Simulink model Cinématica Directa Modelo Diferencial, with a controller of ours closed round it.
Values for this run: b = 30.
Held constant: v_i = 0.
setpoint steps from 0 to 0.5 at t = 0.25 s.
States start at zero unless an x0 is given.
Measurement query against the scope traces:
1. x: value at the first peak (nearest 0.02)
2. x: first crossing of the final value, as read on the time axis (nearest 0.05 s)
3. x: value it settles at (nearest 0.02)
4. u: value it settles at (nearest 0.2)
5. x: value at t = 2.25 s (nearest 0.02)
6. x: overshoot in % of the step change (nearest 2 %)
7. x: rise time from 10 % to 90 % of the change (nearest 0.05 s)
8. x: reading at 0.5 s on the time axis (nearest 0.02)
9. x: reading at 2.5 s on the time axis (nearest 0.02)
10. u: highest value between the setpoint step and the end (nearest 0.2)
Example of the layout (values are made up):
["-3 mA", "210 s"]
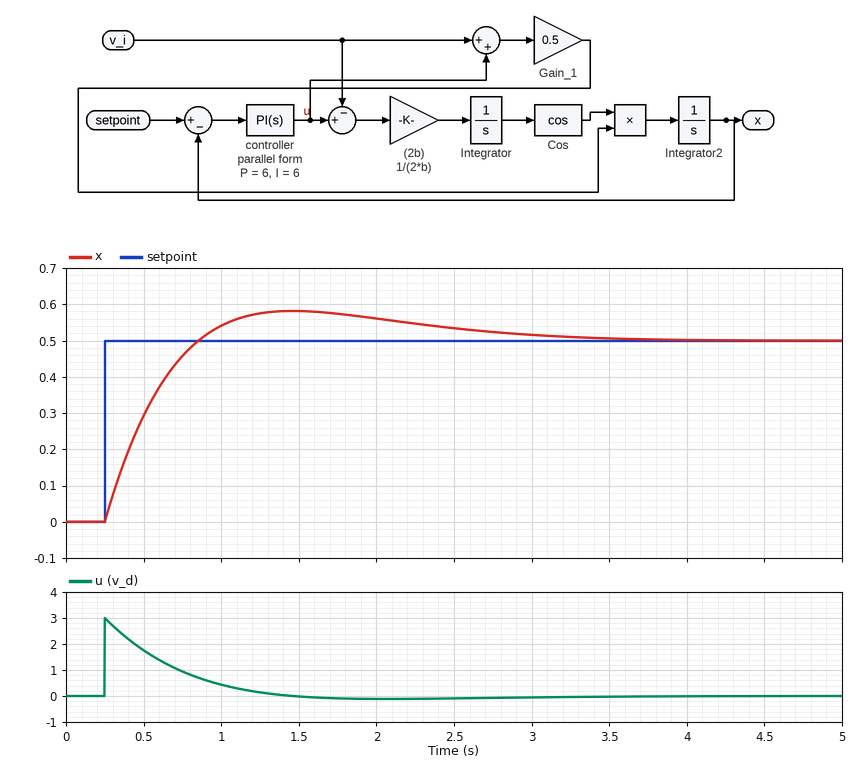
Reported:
["0.58", "0.85 s", "0.50", "0.0", "0.54", "16 %", "0.45 s", "0.30", "0.54", "3.0"]
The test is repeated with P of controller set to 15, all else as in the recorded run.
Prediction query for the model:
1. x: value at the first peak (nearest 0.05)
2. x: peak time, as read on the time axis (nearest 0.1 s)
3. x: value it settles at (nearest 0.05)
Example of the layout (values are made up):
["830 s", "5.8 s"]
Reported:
["0.50", "1.1 s", "0.50"]
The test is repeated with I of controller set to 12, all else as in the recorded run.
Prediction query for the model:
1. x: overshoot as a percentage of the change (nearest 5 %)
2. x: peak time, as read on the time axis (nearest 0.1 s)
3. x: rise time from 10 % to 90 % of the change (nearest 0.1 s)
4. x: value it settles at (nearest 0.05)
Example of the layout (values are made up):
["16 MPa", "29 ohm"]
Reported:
["25 %", "1.2 s", "0.4 s", "0.50"]
